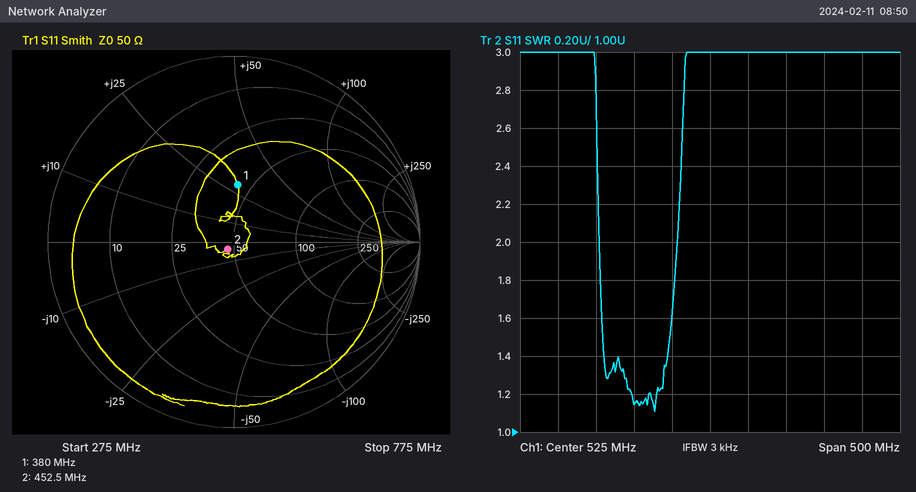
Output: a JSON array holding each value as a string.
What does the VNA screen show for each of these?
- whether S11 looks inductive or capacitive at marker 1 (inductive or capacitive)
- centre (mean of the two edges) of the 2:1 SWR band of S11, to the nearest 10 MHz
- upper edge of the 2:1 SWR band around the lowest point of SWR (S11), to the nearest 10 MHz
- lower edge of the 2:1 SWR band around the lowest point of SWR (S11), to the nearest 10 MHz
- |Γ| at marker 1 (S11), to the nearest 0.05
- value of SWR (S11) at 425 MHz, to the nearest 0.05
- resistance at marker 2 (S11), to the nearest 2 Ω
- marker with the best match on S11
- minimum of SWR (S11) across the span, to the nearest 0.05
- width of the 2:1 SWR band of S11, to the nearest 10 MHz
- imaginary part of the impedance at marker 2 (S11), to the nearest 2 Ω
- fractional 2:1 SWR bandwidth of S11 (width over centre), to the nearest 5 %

["inductive", "430 MHz", "480 MHz", "380 MHz", "0.30", "1.15", "46 Ω", "marker 2", "1.10", "100 MHz", "-4 Ω", "25 %"]
